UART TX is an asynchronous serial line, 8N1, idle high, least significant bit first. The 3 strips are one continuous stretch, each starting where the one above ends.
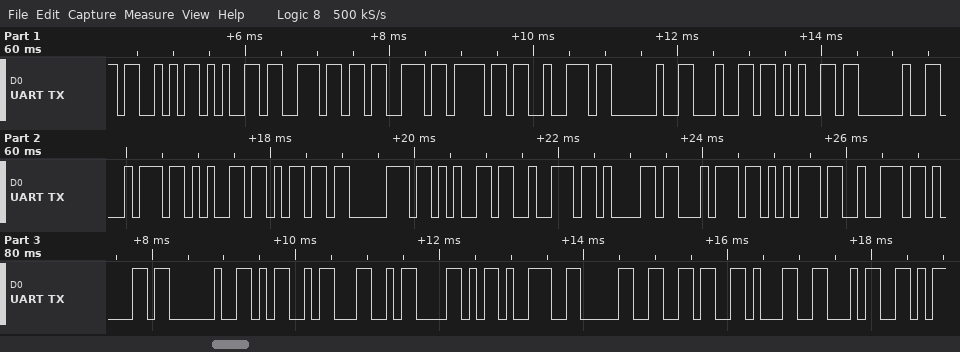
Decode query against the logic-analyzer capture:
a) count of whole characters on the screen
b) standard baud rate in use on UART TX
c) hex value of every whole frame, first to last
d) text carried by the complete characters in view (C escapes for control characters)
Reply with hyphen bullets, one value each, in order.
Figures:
- 30
- 9600 baud
- 53 65 6E 73 6F 72 20 64 65 20 74 65 6D 70 65 72 61 74 75 72 61 20 4D 4C 58 39 30 36 31 34
- "Sensor de temperatura MLX90614"
